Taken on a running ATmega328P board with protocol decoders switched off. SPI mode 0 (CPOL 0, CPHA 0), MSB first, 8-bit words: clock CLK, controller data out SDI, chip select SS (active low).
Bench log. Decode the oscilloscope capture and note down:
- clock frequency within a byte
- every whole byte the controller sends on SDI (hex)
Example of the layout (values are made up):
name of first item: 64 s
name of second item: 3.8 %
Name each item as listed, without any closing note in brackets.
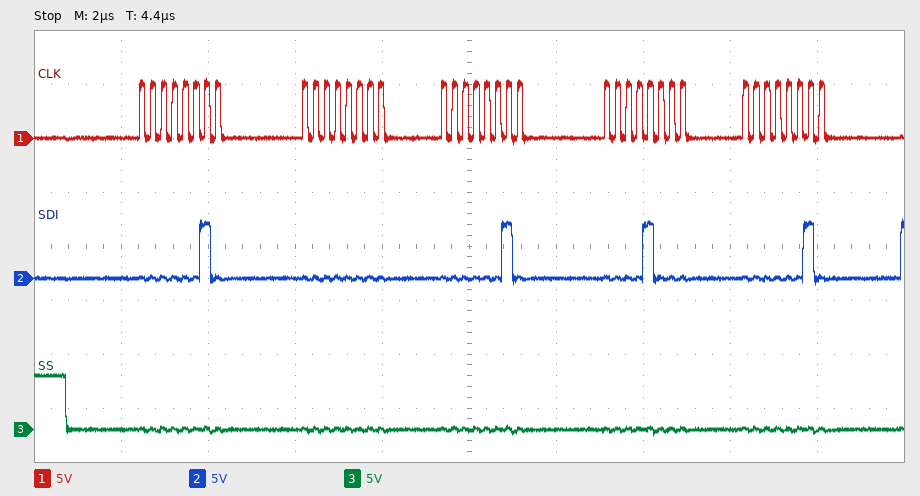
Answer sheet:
clock frequency within a byte: 4 MHz
every whole byte the controller sends on SDI: 0x02 0x00 0x02 0x08 0x02
